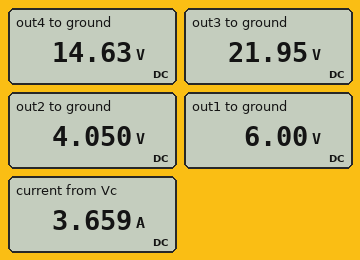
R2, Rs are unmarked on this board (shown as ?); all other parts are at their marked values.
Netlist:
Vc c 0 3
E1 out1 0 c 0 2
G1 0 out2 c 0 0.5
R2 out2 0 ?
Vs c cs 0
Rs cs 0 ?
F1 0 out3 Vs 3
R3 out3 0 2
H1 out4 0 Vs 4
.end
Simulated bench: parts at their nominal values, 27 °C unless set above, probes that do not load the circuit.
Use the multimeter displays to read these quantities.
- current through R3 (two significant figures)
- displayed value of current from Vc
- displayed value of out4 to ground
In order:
11 A
3.659 A
14.63 V
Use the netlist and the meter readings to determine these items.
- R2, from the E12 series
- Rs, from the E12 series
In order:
2.7 Ω
0.82 Ω
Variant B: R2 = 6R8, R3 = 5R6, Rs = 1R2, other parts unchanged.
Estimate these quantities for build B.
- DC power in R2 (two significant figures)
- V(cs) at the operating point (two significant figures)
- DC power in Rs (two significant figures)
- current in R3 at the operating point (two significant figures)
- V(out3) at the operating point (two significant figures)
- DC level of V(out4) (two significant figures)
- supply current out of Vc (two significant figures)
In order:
15 W
3.0 V
7.5 W
7.5 A
42 V
10 V
2.5 A
